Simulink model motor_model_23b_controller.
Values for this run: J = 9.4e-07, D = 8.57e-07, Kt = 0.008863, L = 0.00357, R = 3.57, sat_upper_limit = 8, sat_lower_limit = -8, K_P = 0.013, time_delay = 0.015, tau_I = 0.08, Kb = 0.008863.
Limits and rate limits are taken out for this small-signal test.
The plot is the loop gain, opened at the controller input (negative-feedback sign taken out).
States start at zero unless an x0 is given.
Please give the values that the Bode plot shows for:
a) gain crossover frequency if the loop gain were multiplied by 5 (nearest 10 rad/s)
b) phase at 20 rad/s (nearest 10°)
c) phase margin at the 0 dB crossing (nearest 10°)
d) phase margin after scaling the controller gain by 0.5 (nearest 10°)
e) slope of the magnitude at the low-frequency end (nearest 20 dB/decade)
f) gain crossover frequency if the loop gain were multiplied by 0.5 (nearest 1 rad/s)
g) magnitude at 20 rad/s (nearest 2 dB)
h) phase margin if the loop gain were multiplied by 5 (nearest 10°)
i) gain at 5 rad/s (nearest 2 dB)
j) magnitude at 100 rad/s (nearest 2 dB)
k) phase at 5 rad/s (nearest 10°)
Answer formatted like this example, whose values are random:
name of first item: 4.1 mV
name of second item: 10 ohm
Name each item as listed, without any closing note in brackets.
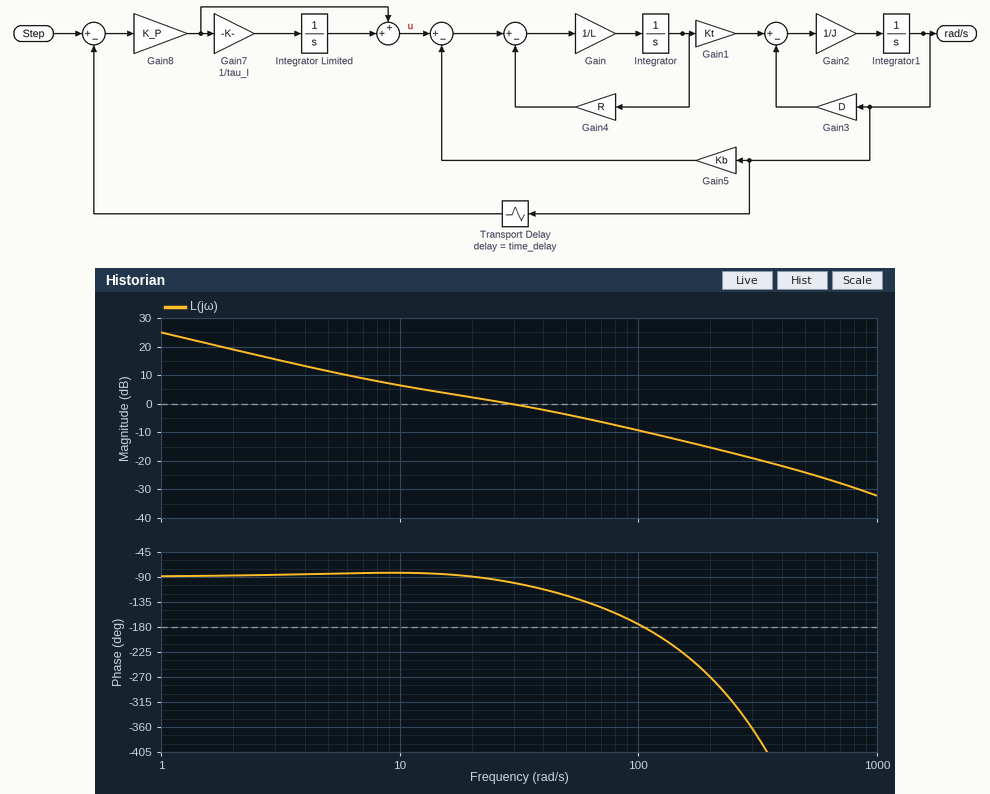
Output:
gain crossover frequency if the loop gain were multiplied by 5: 170 rad/s
phase at 20 rad/s: -90°
phase margin at the 0 dB crossing: 80°
phase margin after scaling the controller gain by 0.5: 100°
slope of the magnitude at the low-frequency end: -20 dB/decade
gain crossover frequency if the loop gain were multiplied by 0.5: 11 rad/s
magnitude at 20 rad/s: 2 dB
phase margin if the loop gain were multiplied by 5: -60°
gain at 5 rad/s: 12 dB
magnitude at 100 rad/s: -10 dB
phase at 5 rad/s: -80°
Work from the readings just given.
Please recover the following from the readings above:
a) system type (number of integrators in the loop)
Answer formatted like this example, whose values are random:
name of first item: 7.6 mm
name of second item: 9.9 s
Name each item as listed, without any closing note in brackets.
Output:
system type: 1
